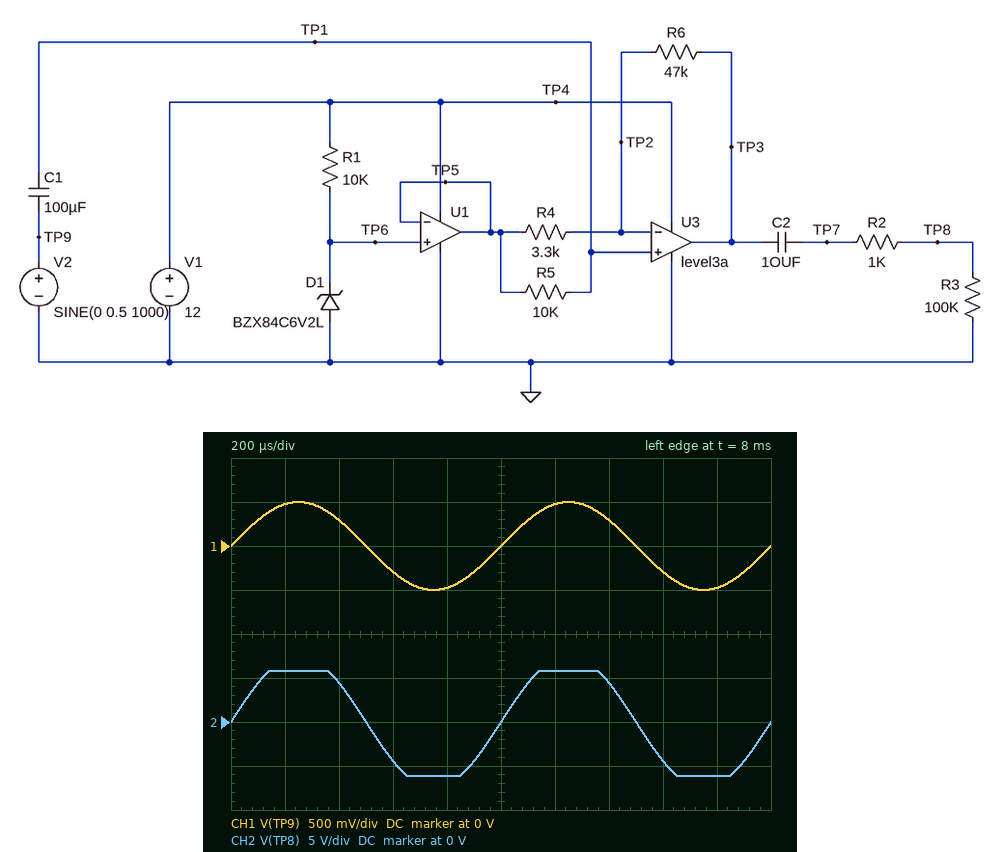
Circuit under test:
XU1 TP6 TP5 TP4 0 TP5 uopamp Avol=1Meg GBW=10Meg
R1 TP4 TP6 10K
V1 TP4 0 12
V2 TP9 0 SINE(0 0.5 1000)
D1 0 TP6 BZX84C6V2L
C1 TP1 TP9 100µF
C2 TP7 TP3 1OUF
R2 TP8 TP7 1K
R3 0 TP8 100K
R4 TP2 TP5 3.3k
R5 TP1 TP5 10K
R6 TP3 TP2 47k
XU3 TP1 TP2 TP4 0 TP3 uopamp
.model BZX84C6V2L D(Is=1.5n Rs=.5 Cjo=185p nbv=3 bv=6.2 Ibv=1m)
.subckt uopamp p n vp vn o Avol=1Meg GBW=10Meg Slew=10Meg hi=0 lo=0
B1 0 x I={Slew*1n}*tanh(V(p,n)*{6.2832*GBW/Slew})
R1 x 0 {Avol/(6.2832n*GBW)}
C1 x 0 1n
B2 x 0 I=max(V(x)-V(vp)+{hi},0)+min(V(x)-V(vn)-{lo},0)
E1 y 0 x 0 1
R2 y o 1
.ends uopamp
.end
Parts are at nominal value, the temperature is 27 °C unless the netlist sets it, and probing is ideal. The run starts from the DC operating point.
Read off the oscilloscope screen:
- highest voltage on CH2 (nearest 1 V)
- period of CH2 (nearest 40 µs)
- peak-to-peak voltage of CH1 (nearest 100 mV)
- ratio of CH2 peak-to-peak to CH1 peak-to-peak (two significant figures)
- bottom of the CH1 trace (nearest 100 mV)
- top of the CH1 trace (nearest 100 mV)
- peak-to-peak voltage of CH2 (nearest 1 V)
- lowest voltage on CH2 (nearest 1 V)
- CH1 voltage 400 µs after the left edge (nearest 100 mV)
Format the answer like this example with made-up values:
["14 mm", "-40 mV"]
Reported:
["6 V", "1.00 ms", "1.0 V", "12", "-500 mV", "500 mV", "12 V", "-6 V", "300 mV"]
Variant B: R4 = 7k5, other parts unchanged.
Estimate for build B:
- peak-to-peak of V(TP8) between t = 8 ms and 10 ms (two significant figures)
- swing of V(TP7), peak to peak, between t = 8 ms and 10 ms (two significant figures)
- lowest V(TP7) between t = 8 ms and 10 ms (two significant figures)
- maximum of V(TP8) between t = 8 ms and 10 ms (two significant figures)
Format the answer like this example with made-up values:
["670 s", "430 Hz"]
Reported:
["7.2 V", "7.3 V", "-3.6 V", "3.6 V"]
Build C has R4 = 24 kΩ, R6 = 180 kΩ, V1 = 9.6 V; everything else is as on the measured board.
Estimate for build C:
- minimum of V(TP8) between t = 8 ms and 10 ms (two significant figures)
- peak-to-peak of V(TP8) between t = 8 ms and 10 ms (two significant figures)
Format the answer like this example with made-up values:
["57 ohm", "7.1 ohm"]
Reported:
["-4.2 V", "7.7 V"]
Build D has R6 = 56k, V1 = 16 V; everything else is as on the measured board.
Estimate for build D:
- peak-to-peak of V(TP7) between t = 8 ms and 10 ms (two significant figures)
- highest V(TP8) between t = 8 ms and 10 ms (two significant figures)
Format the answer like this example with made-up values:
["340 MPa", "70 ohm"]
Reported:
["15 V", "8.9 V"]
